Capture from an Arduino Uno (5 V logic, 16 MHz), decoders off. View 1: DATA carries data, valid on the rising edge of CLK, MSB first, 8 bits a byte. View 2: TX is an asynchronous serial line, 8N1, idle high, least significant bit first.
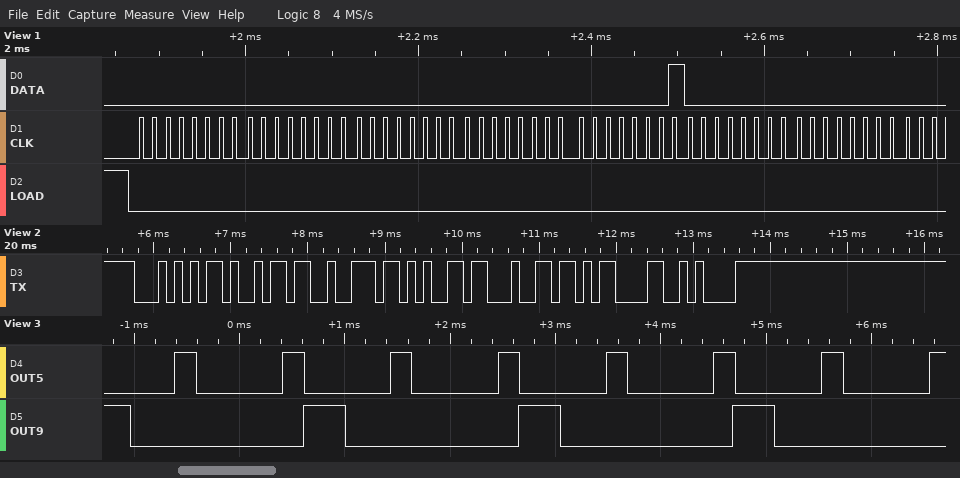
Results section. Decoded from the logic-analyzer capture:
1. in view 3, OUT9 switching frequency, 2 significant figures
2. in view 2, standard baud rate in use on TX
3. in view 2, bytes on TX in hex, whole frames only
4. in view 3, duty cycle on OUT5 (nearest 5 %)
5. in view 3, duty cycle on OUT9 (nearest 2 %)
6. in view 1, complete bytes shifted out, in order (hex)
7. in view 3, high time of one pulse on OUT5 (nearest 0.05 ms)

490 Hz
9600 baud
54 69 72 65 64 0D 0A
20 %
20 %
00 00 00 00 01 00 00
0.20 ms
